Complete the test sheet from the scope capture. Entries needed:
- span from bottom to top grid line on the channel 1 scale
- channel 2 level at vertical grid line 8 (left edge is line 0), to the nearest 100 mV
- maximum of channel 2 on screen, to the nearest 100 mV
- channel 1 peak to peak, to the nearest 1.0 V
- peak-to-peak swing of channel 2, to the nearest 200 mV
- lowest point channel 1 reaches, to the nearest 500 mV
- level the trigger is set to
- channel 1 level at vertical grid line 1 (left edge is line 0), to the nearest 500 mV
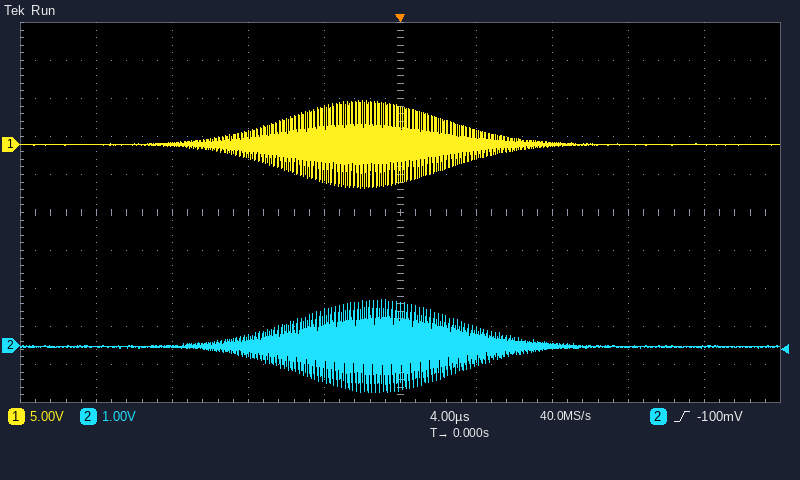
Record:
50 V
0.0 V
1.2 V
12.0 V
2.4 V
-6.0 V
-100 mV
0.0 V
